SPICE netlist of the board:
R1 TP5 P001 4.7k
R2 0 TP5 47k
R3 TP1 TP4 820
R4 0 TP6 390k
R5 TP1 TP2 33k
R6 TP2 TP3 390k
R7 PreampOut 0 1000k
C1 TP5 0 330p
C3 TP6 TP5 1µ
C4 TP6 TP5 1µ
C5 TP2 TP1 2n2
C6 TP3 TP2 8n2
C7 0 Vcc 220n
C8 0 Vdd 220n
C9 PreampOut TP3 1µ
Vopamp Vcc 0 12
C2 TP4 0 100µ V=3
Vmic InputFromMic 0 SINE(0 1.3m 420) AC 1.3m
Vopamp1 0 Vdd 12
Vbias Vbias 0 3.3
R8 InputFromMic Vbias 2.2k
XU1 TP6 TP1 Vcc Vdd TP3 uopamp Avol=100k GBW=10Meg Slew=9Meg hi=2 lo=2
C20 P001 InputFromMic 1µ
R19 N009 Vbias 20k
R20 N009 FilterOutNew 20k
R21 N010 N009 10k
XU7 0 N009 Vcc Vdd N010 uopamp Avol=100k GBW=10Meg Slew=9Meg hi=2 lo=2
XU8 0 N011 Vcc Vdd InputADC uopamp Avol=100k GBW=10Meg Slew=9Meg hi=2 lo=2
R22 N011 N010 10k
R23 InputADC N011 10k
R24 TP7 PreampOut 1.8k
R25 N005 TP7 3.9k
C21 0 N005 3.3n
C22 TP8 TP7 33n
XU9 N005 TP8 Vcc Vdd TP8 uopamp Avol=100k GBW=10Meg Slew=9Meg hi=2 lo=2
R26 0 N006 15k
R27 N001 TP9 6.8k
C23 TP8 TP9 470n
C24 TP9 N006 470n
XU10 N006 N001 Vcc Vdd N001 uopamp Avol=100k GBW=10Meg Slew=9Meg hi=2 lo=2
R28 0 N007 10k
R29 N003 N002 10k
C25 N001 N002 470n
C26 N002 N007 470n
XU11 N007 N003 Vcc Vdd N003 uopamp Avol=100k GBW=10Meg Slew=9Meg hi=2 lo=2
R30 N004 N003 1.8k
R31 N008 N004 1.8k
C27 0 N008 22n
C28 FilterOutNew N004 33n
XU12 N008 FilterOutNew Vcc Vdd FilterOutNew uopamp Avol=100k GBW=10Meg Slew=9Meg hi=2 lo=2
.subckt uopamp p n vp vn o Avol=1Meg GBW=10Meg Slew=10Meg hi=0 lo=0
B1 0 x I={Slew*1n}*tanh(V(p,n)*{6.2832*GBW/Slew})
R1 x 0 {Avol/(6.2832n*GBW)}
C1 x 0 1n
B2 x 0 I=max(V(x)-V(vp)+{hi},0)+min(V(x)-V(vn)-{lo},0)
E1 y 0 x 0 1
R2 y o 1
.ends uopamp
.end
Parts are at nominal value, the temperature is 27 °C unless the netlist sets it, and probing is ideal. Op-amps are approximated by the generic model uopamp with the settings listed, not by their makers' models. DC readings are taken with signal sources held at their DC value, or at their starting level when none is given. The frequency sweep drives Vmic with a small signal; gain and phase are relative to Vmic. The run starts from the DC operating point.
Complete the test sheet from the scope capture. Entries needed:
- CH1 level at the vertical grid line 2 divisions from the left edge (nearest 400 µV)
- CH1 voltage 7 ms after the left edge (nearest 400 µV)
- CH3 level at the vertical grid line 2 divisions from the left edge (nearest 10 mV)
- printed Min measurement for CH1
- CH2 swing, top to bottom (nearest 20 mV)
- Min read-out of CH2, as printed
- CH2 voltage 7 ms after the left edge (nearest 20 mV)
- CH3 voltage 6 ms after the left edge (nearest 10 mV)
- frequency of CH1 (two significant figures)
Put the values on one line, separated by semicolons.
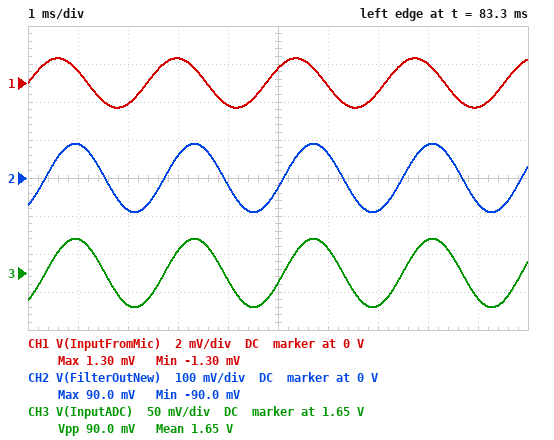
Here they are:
-1.2 mV; -400 µV; 1.61 V; -1.30 mV; 180 mV; -90.0 mV; -80 mV; 1.68 V; 420 Hz
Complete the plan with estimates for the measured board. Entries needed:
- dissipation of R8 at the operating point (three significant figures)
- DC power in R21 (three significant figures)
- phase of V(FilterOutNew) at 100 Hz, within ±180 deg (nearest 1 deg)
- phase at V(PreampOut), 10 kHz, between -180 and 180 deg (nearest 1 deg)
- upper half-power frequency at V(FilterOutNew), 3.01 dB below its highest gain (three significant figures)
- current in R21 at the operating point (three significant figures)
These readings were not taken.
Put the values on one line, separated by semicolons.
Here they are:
4.95 mW; 272 µW; 9 deg; -80 deg; 135 Hz; 165 µA
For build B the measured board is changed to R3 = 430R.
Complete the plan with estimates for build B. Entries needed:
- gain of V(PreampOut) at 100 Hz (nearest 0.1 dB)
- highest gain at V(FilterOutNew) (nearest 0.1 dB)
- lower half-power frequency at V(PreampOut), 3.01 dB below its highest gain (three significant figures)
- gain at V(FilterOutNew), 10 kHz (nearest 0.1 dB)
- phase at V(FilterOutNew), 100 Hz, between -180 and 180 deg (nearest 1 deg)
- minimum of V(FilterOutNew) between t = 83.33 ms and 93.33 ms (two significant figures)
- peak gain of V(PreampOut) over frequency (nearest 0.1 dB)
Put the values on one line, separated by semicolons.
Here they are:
52.0 dB; 52.4 dB; 4.79 Hz; -1.8 dB; 10 deg; -170 mV; 58.0 dB
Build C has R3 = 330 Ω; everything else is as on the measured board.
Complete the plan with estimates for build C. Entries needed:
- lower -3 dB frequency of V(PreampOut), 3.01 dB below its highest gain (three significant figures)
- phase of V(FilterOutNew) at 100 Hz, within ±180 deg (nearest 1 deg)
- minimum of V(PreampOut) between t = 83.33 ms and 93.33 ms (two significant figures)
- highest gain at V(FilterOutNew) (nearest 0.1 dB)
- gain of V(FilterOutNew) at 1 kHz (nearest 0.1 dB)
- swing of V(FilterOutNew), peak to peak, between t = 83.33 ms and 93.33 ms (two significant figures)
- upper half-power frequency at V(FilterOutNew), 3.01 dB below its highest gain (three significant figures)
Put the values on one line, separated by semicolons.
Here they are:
5.44 Hz; 11 deg; -220 mV; 54.7 dB; 41.1 dB; 440 mV; 136 Hz
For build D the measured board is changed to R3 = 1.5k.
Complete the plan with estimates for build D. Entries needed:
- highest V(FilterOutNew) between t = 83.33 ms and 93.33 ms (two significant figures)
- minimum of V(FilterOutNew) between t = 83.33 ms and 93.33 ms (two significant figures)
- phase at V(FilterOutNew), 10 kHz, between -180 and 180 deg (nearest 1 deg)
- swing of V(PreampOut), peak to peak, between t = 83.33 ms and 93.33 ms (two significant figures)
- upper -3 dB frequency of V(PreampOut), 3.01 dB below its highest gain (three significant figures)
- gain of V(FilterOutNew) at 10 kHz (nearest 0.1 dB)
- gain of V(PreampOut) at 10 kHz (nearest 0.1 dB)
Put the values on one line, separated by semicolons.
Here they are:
50 mV; -50 mV; -14 deg; 100 mV; 57.2 Hz; -12.3 dB; 14.8 dB
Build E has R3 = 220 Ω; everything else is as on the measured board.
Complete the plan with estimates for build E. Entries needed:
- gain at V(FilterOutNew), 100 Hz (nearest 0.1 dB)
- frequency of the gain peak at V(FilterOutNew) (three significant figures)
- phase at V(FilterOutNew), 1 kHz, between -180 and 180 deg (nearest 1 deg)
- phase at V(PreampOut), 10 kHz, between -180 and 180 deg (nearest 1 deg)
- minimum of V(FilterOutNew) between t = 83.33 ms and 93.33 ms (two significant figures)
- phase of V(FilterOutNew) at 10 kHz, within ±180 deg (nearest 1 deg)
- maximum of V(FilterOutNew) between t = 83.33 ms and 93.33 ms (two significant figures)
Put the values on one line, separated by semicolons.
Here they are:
56.8 dB; 62.0 Hz; -78 deg; -84 deg; -330 mV; -22 deg; 330 mV
